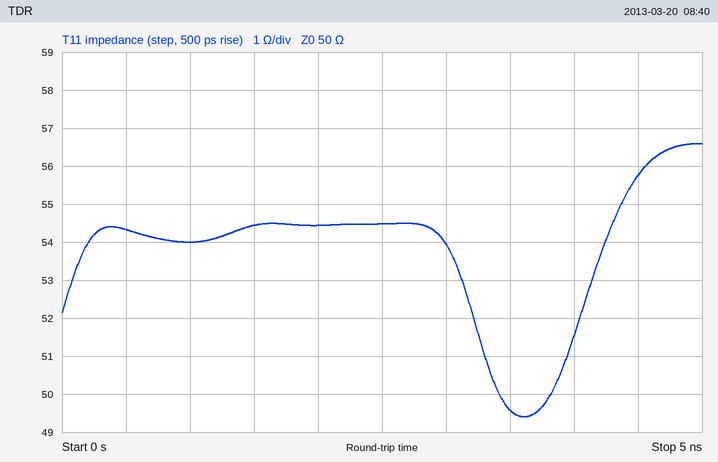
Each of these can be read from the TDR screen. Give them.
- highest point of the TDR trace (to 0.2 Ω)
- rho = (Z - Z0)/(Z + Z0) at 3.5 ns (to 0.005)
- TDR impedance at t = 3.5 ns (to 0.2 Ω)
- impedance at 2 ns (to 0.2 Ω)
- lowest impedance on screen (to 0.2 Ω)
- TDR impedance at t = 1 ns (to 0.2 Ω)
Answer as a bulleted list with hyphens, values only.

- 56.6 Ω
- -0.005
- 49.6 Ω
- 54.4 Ω
- 49.4 Ω
- 54.0 Ω
